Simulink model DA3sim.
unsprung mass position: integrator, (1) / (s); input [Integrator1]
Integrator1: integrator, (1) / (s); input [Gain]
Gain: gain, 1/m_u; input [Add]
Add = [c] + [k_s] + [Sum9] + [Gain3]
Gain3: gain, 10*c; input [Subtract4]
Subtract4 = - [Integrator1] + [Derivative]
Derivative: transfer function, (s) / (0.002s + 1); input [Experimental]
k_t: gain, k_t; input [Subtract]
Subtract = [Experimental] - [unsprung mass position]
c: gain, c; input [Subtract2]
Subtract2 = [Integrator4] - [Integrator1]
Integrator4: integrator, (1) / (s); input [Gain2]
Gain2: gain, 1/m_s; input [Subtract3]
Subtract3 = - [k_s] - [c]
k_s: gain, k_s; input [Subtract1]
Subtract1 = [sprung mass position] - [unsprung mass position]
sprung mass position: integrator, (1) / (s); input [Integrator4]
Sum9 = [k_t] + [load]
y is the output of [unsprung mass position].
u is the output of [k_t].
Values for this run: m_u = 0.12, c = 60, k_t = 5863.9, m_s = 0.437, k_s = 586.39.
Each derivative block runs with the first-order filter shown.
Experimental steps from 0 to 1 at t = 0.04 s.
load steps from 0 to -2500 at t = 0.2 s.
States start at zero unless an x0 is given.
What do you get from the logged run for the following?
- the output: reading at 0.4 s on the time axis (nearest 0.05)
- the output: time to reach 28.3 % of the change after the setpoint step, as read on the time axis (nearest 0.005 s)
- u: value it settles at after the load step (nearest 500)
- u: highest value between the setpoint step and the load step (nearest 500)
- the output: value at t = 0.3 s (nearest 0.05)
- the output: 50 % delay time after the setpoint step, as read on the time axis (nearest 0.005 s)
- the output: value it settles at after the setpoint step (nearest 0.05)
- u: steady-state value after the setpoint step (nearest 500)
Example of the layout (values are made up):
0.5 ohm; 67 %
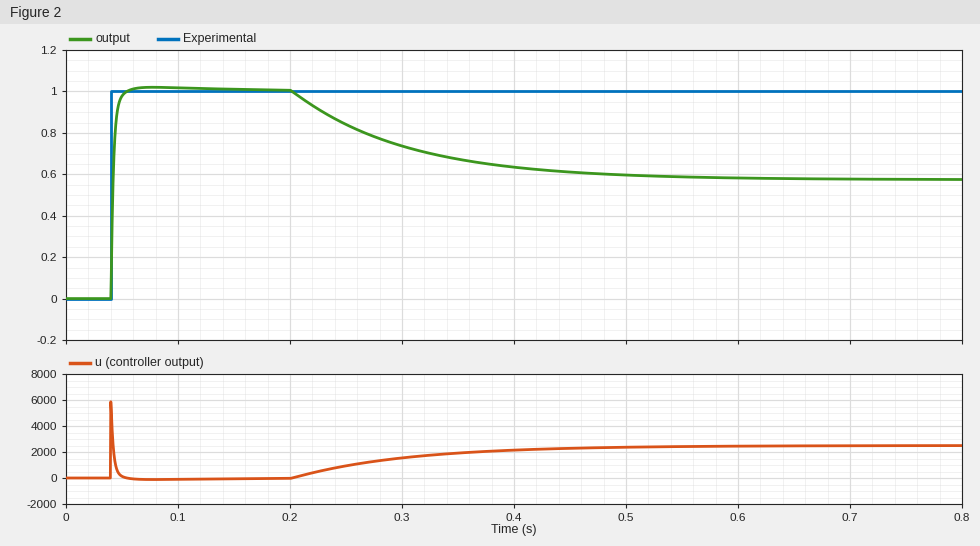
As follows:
0.65; 0.040 s; 2500; 6000; 0.75; 0.040 s; 1.00; 0
